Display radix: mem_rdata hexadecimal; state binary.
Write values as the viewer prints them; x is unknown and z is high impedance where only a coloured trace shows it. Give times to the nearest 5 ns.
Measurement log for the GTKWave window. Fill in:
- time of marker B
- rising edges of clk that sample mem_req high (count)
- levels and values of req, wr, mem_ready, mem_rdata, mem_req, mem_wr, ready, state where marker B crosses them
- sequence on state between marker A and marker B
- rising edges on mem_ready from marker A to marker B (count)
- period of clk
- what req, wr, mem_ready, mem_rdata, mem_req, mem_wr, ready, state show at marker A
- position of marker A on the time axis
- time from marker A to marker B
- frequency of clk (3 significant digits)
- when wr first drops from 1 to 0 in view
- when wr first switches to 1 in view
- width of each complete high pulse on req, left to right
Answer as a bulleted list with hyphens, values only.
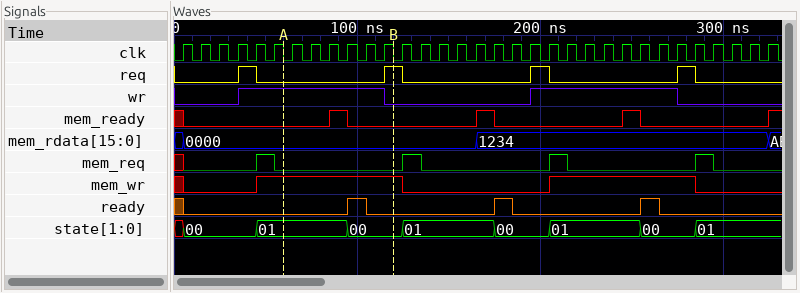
- 120 ns
- 4
- req=1, wr=0, mem_ready=0, mem_rdata=0000, mem_req=0, mem_wr=1, ready=0, state=00
- 01, 00
- 1
- 10 ns
- req=0, wr=1, mem_ready=0, mem_rdata=0000, mem_req=0, mem_wr=1, ready=0, state=01
- 60 ns
- 60 ns
- 100 MHz
- 115 ns
- 35 ns
- 10 ns, 10 ns, 10 ns, 10 ns
